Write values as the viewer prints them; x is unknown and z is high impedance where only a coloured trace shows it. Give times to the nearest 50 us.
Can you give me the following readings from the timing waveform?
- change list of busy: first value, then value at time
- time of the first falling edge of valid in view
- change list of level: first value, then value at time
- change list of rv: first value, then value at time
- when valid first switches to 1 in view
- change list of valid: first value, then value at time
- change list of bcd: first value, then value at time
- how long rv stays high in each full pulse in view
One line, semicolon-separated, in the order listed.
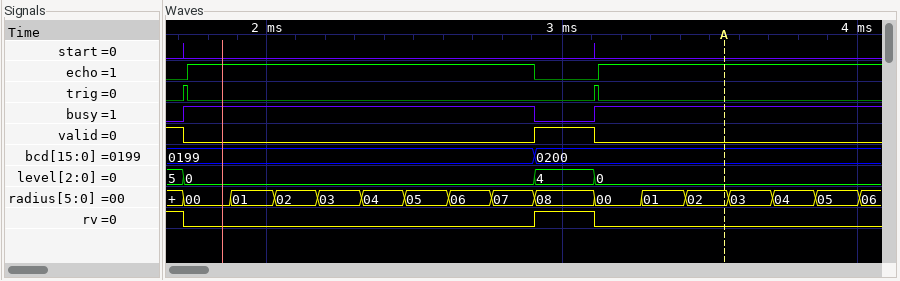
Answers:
0, 1 at 1700 us, 0 at 2900 us, 1 at 3100 us; 1700 us; 5, 0 at 1700 us, 4 at 2900 us, 0 at 3100 us; 1, 0 at 1700 us, 1 at 2900 us, 0 at 3100 us; 2900 us; 1, 0 at 1700 us, 1 at 2900 us, 0 at 3100 us; 0199, 0200 at 2900 us; 200 us
